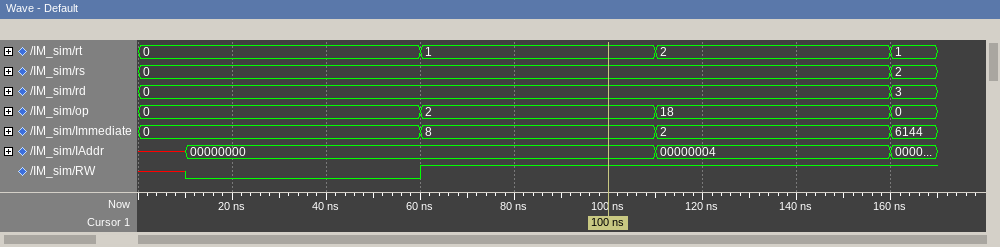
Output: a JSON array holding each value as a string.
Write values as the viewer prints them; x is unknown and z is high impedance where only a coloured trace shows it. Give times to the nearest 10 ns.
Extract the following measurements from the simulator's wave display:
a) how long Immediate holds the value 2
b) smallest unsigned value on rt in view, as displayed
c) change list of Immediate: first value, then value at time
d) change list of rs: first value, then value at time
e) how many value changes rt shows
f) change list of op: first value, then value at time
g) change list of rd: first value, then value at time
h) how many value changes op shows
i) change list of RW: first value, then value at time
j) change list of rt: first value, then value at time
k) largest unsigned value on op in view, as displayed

["50 ns", "0", "0, 8 at 60 ns, 2 at 110 ns, 6144 at 160 ns", "0, 2 at 160 ns", "3", "0, 2 at 60 ns, 18 at 110 ns, 0 at 160 ns", "0, 3 at 160 ns", "3", "x, 0 at 10 ns, 1 at 60 ns", "0, 1 at 60 ns, 2 at 110 ns, 1 at 160 ns", "18"]
